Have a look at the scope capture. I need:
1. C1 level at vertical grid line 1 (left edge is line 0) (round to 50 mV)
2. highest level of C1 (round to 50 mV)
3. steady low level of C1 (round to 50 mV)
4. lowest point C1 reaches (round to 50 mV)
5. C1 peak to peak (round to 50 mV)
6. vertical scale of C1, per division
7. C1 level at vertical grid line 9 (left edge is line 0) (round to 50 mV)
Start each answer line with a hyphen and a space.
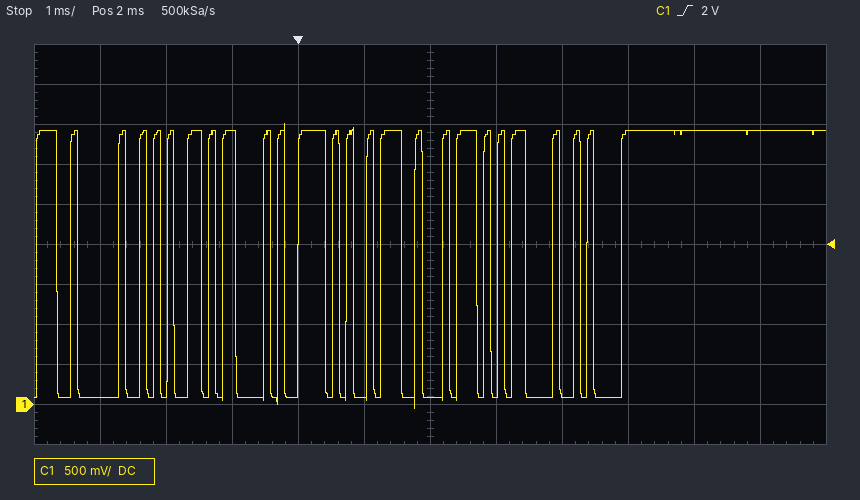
- 100 mV
- 3.50 V
- 100 mV
- -50 mV
- 3.55 V
- 500 mV
- 3.40 V
